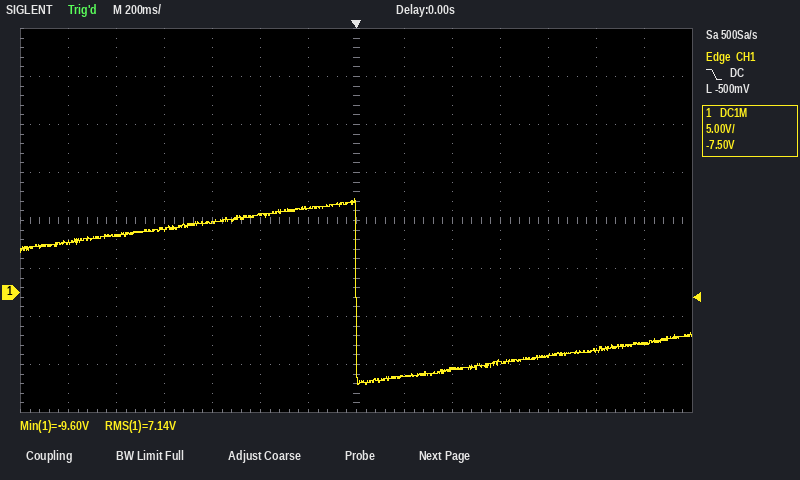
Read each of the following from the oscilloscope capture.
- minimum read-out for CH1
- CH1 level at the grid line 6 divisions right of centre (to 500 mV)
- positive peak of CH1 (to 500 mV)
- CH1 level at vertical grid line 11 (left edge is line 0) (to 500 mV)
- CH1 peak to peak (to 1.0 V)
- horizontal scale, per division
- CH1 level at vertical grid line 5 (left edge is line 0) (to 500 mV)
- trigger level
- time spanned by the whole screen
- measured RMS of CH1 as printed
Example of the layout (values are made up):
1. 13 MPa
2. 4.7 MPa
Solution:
1. -9.60 V
2. -5.5 V
3. 10.0 V
4. -6.5 V
5. 19.0 V
6. 200 ms
7. 8.0 V
8. -500 mV
9. 2.8 s
10. 7.14 V
